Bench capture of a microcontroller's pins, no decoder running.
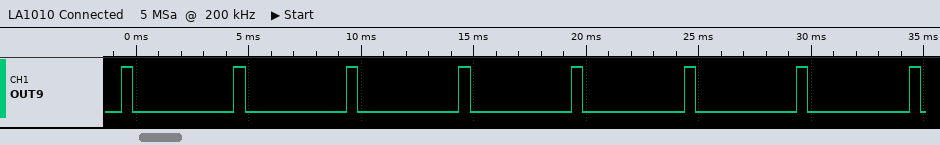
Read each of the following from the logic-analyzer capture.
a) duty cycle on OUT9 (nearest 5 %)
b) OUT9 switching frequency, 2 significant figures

10 %
200 Hz
